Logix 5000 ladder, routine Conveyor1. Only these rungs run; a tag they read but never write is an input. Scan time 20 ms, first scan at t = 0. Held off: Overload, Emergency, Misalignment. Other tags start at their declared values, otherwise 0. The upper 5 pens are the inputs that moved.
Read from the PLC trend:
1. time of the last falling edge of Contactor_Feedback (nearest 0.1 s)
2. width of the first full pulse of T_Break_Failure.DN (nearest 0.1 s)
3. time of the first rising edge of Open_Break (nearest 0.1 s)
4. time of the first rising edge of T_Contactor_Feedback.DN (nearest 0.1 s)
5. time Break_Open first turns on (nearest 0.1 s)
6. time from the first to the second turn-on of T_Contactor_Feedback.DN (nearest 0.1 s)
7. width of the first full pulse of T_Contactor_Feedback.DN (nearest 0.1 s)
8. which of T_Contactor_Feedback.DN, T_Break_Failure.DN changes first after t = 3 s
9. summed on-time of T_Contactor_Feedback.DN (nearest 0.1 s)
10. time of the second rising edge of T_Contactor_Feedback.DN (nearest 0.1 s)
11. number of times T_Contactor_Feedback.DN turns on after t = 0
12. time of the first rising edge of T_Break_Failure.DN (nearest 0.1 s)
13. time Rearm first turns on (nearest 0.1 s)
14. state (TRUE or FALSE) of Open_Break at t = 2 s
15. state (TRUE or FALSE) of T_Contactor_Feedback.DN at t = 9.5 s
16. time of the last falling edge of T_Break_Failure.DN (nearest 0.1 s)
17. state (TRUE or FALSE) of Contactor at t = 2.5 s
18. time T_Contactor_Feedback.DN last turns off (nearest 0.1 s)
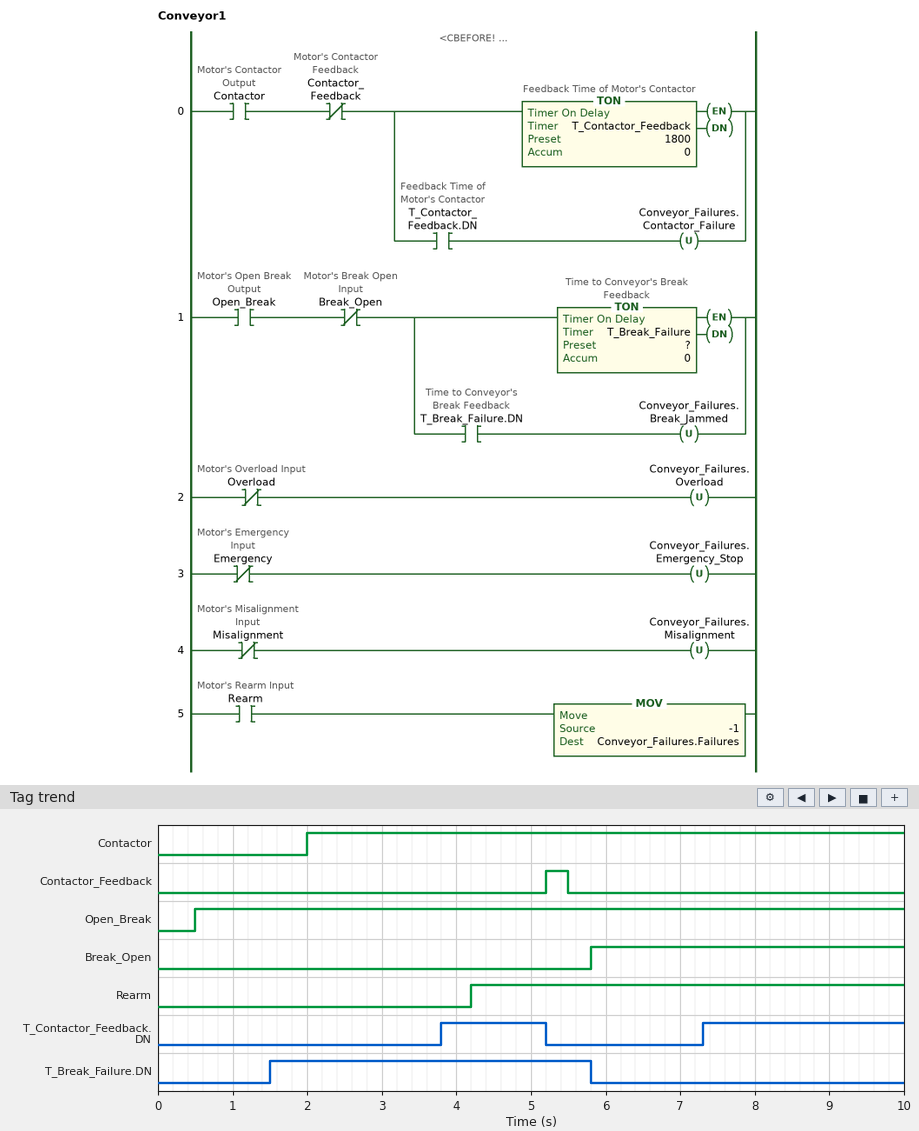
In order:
5.5 s
4.3 s
0.5 s
3.8 s
5.8 s
3.5 s
1.4 s
T_Contactor_Feedback.DN
4.1 s
7.3 s
2
1.5 s
4.2 s
TRUE
TRUE
5.8 s
TRUE
5.2 s
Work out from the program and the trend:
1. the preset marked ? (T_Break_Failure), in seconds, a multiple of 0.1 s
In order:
1.0 s
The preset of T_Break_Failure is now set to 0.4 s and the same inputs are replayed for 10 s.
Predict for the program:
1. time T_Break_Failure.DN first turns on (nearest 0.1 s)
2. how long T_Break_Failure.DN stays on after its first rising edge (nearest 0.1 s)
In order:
0.9 s
4.9 s
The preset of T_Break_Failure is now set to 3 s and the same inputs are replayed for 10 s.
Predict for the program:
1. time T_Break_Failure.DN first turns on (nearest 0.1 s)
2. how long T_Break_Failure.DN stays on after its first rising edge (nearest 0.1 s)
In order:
3.5 s
2.3 s
